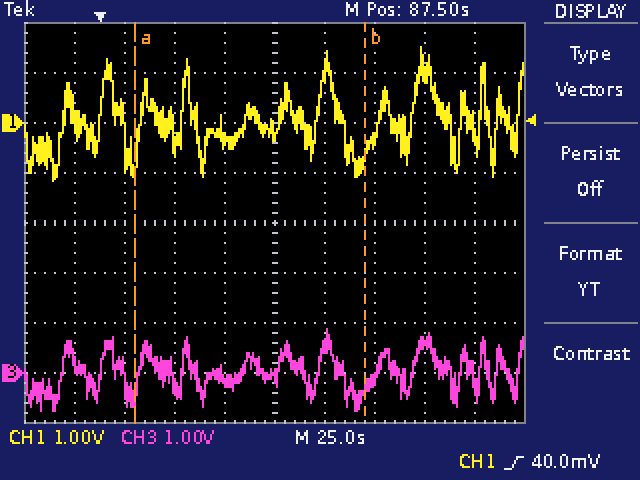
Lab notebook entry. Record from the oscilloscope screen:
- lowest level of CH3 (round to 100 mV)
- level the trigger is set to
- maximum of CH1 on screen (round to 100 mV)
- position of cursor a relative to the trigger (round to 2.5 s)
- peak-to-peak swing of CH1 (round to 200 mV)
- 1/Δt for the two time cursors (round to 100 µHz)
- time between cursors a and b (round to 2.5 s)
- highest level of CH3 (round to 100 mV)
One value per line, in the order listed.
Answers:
-800 mV
40.0 mV
1.5 V
+17.5 s
2.6 V
8.7 mHz
115.0 s
900 mV
